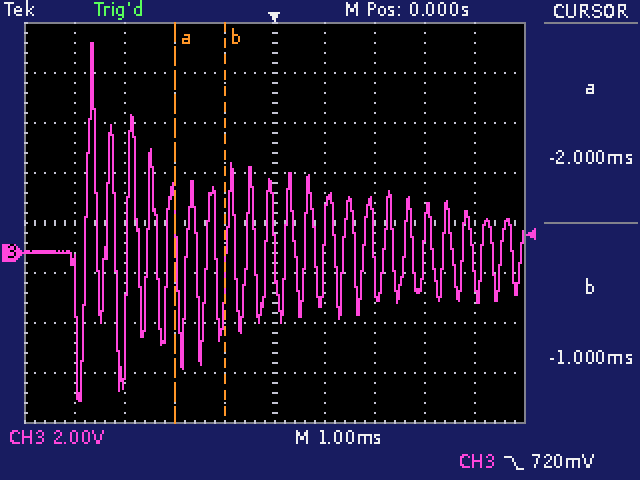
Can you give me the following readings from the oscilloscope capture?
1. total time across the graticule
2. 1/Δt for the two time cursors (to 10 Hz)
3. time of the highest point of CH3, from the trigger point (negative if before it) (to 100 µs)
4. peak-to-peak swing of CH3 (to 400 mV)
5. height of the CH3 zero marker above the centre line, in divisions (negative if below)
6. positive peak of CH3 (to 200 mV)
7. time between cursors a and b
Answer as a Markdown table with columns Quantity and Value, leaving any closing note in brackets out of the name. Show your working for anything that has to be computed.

| Quantity | Value |
|---|---|
| total time across the graticule | 10 ms |
| 1/Δt for the two time cursors | 1 / 1.0 ms ≈ 1.00 kHz |
| time of the highest point of CH3, from the trigger point (negative if before it) | -3.6 ms |
| peak-to-peak swing of CH3 | 14.4 V |
| height of the CH3 zero marker above the centre line, in divisions | -0.6 div |
| positive peak of CH3 | 8.4 V |
| time between cursors a and b | -1 ms − (-2 ms) = 1.0 ms |
